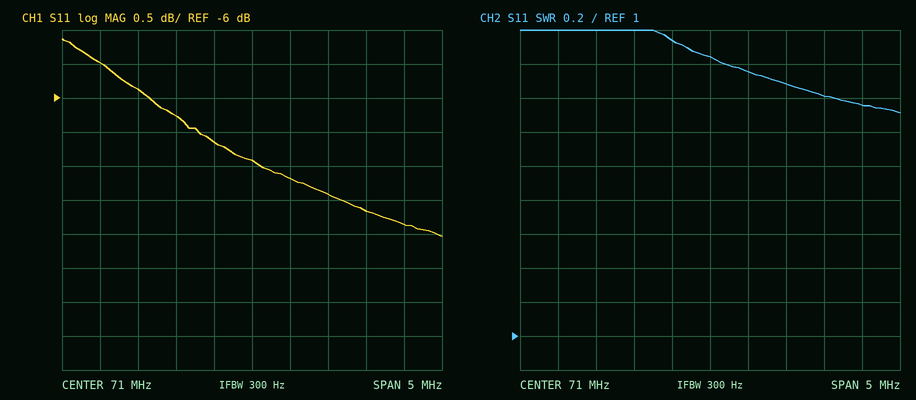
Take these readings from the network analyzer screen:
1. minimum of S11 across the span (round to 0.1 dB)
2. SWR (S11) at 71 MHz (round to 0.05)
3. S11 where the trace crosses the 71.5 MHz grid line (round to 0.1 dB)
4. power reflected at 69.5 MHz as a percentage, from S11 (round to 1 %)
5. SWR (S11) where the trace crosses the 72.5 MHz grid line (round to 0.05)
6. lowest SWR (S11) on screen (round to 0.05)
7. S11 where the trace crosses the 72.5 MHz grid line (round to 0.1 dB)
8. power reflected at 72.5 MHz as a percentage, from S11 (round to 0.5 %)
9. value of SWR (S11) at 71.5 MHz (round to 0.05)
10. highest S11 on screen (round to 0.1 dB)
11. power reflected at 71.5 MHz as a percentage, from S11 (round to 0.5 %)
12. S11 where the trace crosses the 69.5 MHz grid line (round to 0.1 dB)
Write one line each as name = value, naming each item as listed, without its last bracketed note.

minimum of S11 across the span = -8.0 dB
SWR (S11) at 71 MHz = 2.65
S11 where the trace crosses the 71.5 MHz grid line = -7.2 dB
power reflected at 69.5 MHz as a percentage, from S11 = 26 %
SWR (S11) where the trace crosses the 72.5 MHz grid line = 2.40
lowest SWR (S11) on screen = 2.30
S11 where the trace crosses the 72.5 MHz grid line = -7.7 dB
power reflected at 72.5 MHz as a percentage, from S11 = 17.0 %
value of SWR (S11) at 71.5 MHz = 2.55
highest S11 on screen = -5.1 dB
power reflected at 71.5 MHz as a percentage, from S11 = 19.0 %
S11 where the trace crosses the 69.5 MHz grid line = -5.9 dB
